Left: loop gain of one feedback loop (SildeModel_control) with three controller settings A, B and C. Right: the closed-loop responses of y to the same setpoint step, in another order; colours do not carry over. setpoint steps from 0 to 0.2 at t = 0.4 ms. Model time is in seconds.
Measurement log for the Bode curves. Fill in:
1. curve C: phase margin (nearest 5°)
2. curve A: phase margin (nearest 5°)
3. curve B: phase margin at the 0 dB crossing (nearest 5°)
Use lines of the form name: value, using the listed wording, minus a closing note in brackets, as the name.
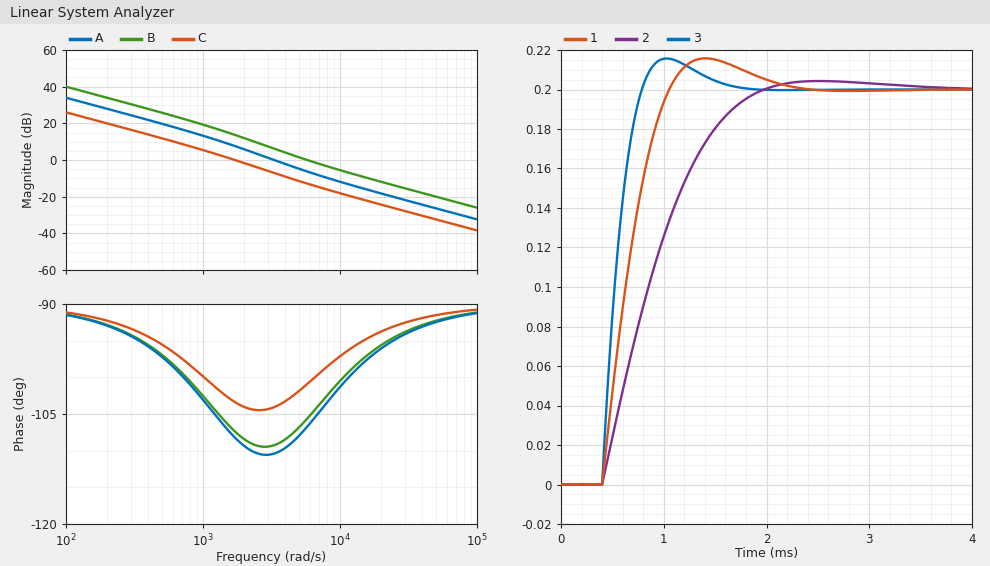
curve C: phase margin: 75°
curve A: phase margin: 70°
curve B: phase margin at the 0 dB crossing: 75°
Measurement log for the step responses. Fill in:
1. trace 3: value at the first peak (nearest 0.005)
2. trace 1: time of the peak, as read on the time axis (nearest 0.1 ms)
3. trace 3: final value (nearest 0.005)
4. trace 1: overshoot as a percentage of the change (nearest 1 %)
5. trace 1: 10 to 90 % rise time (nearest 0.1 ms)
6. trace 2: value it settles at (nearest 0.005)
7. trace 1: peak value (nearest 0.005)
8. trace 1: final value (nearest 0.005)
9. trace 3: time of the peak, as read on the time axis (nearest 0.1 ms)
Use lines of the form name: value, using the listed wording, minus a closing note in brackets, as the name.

trace 3: value at the first peak: 0.215
trace 1: time of the peak, as read on the time axis: 1.4 ms
trace 3: final value: 0.200
trace 1: overshoot as a percentage of the change: 8 %
trace 1: 10 to 90 % rise time: 0.5 ms
trace 2: value it settles at: 0.200
trace 1: peak value: 0.215
trace 1: final value: 0.200
trace 3: time of the peak, as read on the time axis: 1.0 ms
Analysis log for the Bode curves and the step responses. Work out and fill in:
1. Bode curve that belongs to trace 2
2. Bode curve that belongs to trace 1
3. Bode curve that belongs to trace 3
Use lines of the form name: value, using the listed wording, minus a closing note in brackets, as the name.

Bode curve that belongs to trace 2: C
Bode curve that belongs to trace 1: A
Bode curve that belongs to trace 3: B
